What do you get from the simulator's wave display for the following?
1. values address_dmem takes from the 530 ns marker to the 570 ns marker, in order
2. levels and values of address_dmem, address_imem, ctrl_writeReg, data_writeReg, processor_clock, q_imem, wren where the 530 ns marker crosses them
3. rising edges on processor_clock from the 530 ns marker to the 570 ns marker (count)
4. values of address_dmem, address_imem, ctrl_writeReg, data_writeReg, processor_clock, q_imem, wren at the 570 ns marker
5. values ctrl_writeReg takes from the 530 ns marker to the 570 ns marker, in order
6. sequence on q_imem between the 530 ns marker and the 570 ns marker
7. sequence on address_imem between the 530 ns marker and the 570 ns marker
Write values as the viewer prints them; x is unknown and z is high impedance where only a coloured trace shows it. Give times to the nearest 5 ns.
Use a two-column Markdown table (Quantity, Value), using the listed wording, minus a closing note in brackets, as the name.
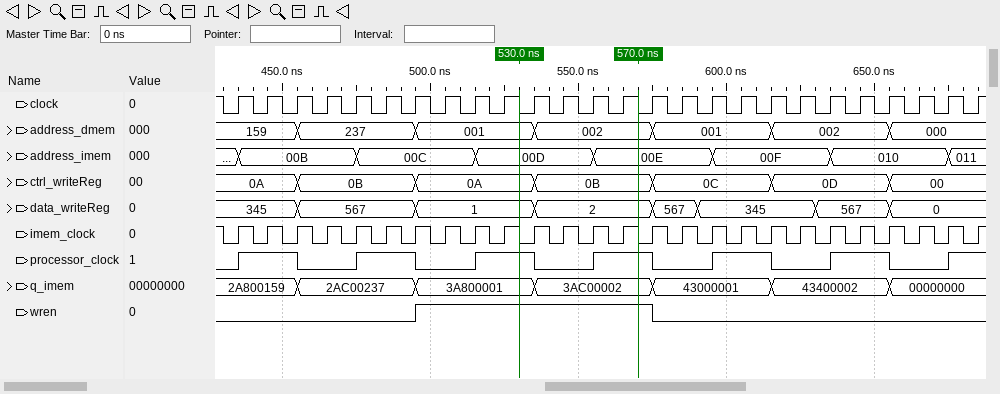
| Quantity | Value |
|---|---|
| values address_dmem takes from the 530 ns marker to the 570 ns marker, in order | 001, 002 |
| levels and values of address_dmem, address_imem, ctrl_writeReg, data_writeReg, processor_clock, q_imem, wren where the 530 ns marker crosses them | address_dmem=001, address_imem=00D, ctrl_writeReg=0A, data_writeReg=1, processor_clock=1, q_imem=3A800001, wren=1 |
| rising edges on processor_clock from the 530 ns marker to the 570 ns marker | 1 |
| values of address_dmem, address_imem, ctrl_writeReg, data_writeReg, processor_clock, q_imem, wren at the 570 ns marker | address_dmem=002, address_imem=00E, ctrl_writeReg=0B, data_writeReg=2, processor_clock=1, q_imem=3AC00002, wren=1 |
| values ctrl_writeReg takes from the 530 ns marker to the 570 ns marker, in order | 0A, 0B |
| sequence on q_imem between the 530 ns marker and the 570 ns marker | 3A800001, 3AC00002 |
| sequence on address_imem between the 530 ns marker and the 570 ns marker | 00D, 00E |
